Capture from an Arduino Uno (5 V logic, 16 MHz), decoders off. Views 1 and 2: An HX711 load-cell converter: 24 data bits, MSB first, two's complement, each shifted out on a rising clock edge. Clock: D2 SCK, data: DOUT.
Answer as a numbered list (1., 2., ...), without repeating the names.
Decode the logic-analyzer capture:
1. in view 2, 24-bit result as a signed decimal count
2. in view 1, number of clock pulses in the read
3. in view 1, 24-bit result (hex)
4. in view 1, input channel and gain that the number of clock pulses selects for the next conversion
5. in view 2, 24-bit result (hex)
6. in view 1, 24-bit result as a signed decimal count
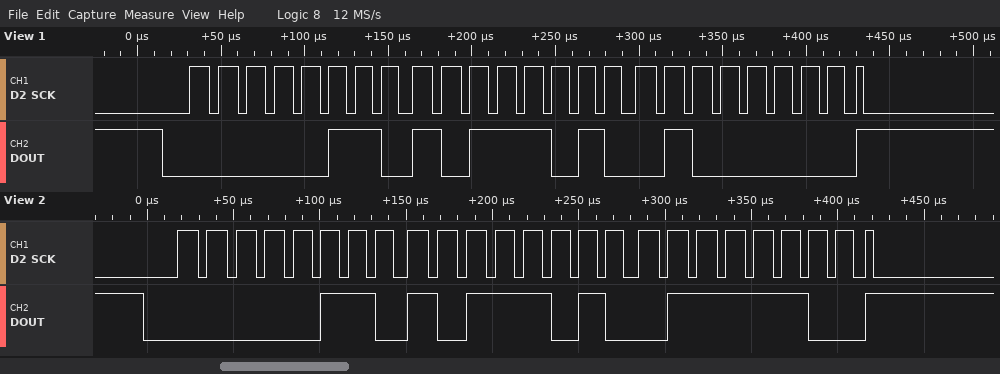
1. 440956
2. 25
3. 0x06BA40
4. channel A, gain 128
5. 0x06BA7C
6. 440896
